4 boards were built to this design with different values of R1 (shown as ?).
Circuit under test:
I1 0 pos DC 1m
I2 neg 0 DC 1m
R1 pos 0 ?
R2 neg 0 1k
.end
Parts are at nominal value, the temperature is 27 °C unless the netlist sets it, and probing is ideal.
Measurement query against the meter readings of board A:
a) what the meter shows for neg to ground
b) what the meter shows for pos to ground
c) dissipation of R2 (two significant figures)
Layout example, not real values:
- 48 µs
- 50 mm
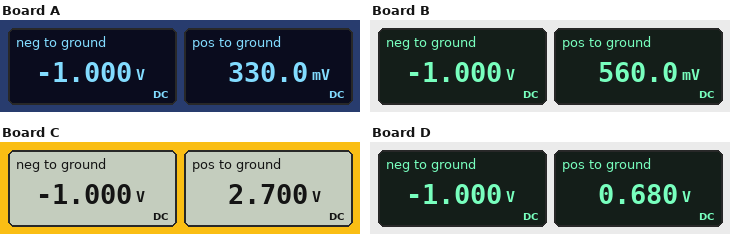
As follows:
- -1.000 V
- 330.0 mV
- 1.0 mW
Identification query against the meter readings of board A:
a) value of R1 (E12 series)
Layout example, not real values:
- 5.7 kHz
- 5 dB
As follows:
- 330 Ω
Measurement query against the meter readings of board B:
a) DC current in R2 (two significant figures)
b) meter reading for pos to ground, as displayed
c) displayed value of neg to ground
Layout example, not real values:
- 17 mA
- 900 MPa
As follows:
- 1.0 mA
- 560.0 mV
- -1.000 V
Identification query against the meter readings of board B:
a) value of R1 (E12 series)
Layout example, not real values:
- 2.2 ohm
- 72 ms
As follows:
- 560 Ω
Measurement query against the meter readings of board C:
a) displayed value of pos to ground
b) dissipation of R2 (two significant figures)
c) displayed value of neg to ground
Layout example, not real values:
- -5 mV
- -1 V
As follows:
- 2.700 V
- 1.0 mW
- -1.000 V
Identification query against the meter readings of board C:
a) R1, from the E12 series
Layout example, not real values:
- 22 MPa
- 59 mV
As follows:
- 2.7 kΩ
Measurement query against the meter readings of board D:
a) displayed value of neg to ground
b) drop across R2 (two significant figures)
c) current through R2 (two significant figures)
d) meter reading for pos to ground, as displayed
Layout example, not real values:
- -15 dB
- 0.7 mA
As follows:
- -1.000 V
- 1.0 V
- 1.0 mA
- 0.680 V
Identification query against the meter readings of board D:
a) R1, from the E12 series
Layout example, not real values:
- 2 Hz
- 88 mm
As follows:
- 680 Ω
